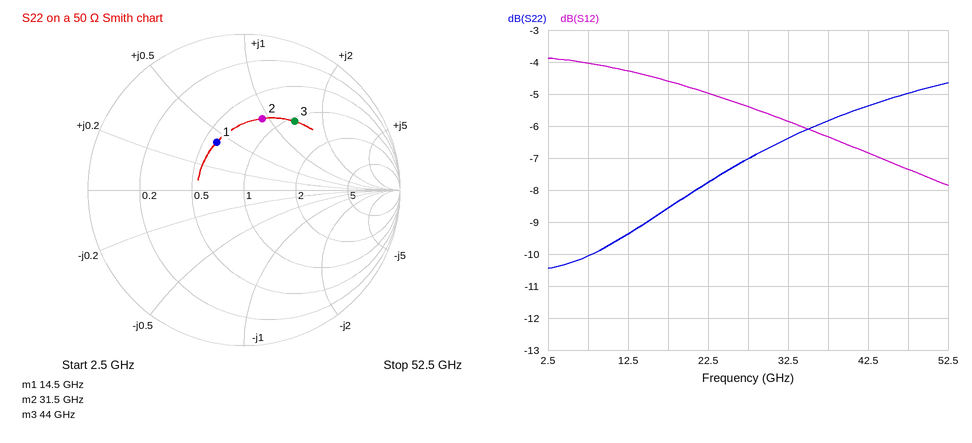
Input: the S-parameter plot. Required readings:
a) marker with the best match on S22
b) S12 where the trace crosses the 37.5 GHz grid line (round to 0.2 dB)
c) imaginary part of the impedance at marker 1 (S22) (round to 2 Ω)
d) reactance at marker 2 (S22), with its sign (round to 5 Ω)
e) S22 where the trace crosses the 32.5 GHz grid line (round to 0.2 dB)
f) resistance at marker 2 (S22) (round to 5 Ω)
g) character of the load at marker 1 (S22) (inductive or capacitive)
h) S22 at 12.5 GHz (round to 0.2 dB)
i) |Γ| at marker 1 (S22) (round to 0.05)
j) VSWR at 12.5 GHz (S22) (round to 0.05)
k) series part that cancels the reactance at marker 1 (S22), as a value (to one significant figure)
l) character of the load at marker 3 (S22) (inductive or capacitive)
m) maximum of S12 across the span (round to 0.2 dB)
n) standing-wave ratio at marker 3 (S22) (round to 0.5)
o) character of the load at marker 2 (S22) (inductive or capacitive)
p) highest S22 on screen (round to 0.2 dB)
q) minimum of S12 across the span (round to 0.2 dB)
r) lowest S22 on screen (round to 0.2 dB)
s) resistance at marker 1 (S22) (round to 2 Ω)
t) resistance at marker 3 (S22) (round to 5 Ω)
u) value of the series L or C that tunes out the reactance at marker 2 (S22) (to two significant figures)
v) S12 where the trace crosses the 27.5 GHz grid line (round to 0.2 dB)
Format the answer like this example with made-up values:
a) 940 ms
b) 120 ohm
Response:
a) marker 1
b) -6.4 dB
c) +20 Ω
d) +45 Ω
e) -6.4 dB
f) 40 Ω
g) inductive
h) -9.4 dB
i) 0.35
j) 2.05
k) 500 fF
l) inductive
m) -3.8 dB
n) 3.5
o) inductive
p) -4.6 dB
q) -7.8 dB
r) -10.4 dB
s) 30 Ω
t) 55 Ω
u) 110 fF
v) -5.4 dB
